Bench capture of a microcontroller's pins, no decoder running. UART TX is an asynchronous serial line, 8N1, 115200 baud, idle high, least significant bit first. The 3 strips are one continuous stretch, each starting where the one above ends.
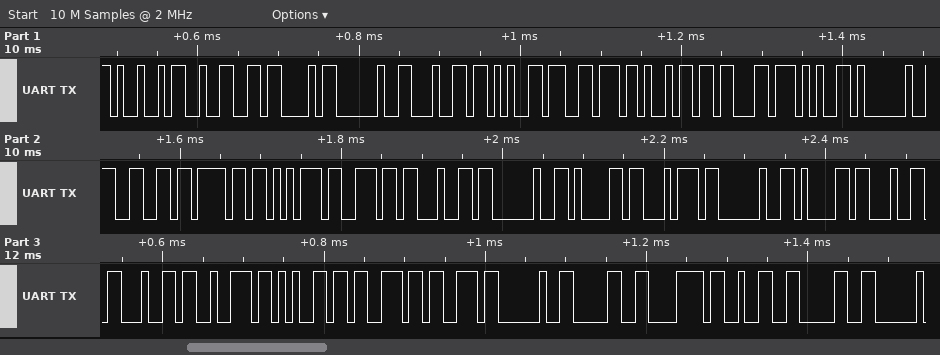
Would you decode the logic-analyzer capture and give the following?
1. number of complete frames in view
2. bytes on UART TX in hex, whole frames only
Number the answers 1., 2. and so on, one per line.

1. 32
2. 0x49 0x32 0x43 0x20 0x64 0x65 0x76 0x69 0x63 0x65 0x20 0x66 0x6F 0x75 0x6E 0x64 0x20 0x61 0x74 0x20 0x61 0x64 0x64 0x72 0x65 0x73 0x73 0x20 0x30 0x78 0x32 0x30
